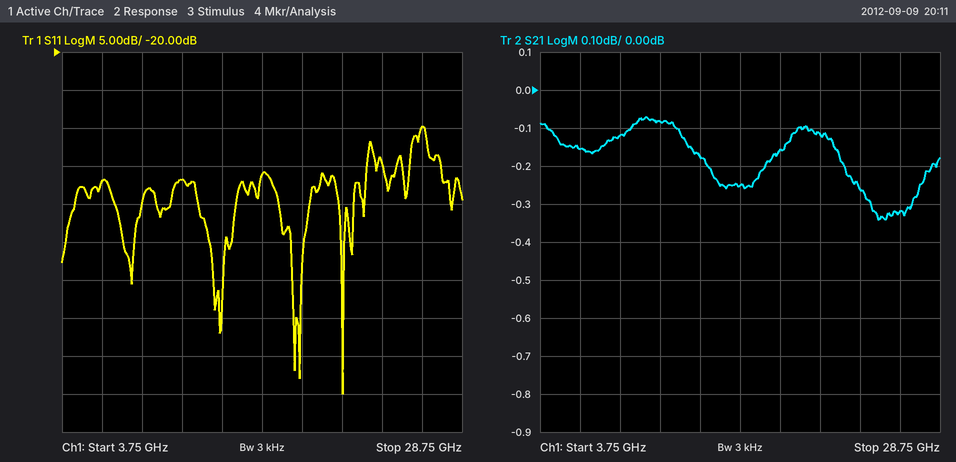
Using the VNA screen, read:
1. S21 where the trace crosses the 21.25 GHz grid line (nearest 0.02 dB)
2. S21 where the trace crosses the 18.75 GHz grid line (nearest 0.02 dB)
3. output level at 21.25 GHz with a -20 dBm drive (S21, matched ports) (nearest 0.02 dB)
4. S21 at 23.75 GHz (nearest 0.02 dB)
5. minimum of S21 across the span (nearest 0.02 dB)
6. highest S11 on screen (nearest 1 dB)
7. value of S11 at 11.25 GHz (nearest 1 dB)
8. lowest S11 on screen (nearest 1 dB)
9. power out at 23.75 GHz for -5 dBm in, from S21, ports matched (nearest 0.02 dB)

-0.12 dB
-0.16 dB
-20.12 dBm
-0.26 dB
-0.34 dB
-30 dB
-37 dB
-65 dB
-5.26 dBm
